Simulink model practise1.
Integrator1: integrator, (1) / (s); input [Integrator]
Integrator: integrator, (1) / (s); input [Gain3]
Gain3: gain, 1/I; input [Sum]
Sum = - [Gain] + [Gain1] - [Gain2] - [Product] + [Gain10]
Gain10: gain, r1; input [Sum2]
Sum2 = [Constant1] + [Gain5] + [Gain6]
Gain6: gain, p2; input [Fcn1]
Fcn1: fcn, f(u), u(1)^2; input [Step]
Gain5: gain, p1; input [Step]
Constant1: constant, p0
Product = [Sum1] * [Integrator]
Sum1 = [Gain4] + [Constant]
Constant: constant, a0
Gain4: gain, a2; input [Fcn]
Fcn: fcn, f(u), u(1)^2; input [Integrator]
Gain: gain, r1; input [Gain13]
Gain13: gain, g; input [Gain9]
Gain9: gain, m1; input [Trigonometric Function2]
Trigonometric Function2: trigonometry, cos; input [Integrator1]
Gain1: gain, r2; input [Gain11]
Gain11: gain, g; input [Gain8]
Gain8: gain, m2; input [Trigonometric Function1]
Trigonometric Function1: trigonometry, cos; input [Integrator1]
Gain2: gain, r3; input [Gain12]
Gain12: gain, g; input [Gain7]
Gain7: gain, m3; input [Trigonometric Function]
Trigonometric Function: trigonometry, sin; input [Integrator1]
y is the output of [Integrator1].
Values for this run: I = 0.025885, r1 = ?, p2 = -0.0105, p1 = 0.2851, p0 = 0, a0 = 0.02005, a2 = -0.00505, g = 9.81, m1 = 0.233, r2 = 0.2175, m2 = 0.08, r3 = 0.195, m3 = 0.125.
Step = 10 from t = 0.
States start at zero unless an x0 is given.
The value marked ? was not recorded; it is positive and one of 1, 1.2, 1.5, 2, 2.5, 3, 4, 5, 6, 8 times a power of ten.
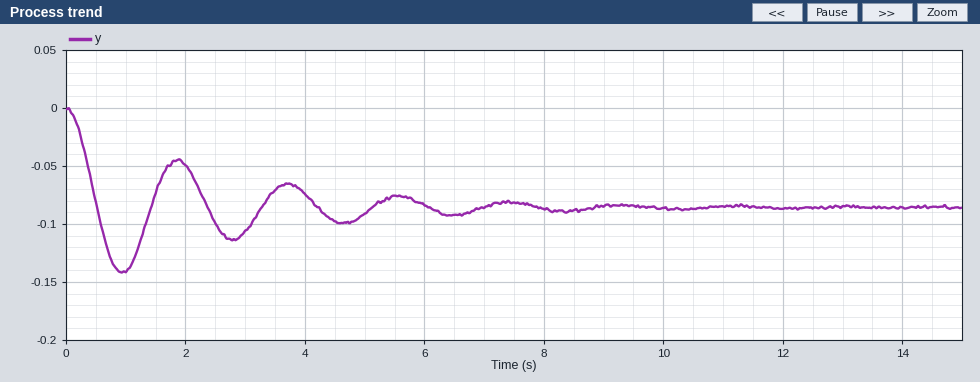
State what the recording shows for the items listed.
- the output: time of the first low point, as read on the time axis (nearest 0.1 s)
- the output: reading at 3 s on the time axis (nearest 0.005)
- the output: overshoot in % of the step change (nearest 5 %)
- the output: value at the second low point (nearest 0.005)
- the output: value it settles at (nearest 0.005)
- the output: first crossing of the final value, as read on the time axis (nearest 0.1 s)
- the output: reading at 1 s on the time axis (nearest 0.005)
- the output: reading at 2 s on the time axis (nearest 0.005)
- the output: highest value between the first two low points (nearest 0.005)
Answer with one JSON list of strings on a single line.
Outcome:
["0.9 s", "-0.105", "65 %", "-0.115", "-0.085", "0.5 s", "-0.140", "-0.050", "-0.045"]
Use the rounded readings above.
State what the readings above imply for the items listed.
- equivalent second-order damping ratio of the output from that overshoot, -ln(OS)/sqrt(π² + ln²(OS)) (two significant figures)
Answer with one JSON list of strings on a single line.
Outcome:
["0.14"]
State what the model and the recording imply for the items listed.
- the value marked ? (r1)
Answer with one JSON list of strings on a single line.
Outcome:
["0.4"]
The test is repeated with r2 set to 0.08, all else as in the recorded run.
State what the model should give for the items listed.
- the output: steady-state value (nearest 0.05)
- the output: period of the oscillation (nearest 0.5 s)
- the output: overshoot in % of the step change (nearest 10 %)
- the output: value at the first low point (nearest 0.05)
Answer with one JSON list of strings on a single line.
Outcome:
["-0.35", "1.5 s", "70 %", "-0.60"]
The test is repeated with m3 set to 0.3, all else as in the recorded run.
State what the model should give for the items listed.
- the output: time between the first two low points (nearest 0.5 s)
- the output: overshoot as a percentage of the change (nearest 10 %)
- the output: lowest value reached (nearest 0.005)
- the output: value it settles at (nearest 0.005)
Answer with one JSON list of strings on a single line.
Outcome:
["1.5 s", "80 %", "-0.070", "-0.040"]
